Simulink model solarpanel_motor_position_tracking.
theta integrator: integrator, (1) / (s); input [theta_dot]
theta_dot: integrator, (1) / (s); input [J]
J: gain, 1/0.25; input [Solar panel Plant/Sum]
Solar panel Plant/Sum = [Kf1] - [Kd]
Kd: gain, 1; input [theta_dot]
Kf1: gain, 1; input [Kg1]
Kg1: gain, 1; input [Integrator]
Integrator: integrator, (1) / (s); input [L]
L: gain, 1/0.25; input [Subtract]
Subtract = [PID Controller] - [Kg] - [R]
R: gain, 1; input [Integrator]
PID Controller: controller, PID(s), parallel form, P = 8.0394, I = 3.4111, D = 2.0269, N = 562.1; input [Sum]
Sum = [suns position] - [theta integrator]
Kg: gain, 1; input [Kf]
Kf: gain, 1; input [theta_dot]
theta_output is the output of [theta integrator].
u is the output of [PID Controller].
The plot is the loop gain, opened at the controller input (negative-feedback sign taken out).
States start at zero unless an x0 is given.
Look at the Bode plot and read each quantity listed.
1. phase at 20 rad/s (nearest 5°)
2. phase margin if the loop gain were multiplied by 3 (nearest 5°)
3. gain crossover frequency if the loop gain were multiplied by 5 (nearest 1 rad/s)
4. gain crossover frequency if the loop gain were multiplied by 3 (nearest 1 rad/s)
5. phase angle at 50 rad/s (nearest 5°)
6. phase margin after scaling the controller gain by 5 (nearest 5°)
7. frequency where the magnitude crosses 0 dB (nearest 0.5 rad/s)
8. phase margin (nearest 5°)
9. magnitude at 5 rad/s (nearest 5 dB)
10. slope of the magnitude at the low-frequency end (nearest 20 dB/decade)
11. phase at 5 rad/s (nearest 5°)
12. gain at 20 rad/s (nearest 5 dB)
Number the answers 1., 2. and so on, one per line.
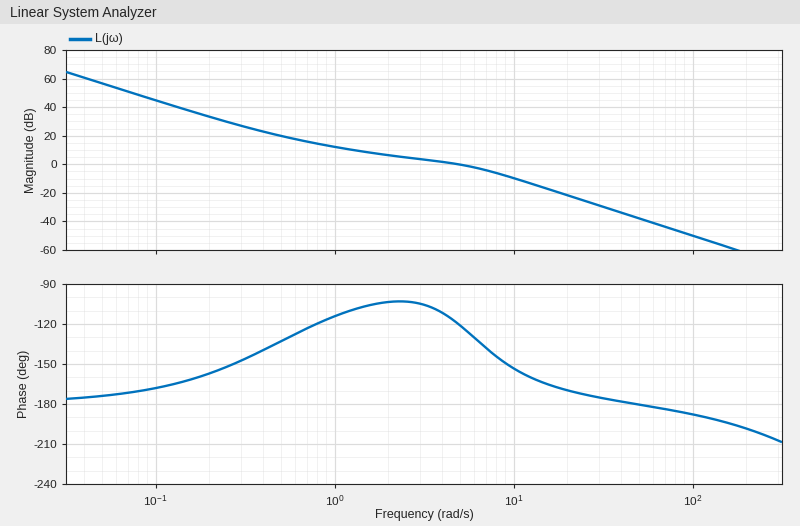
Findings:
1. -170°
2. 25°
3. 13 rad/s
4. 10 rad/s
5. -180°
6. 20°
7. 5.0 rad/s
8. 60°
9. 0 dB
10. -40 dB/decade
11. -120°
12. -20 dB
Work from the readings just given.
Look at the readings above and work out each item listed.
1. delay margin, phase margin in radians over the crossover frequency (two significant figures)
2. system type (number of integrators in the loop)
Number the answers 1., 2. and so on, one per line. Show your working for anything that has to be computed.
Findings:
1. 60 × π / 180 / 5 = 0.21 s
2. 2
